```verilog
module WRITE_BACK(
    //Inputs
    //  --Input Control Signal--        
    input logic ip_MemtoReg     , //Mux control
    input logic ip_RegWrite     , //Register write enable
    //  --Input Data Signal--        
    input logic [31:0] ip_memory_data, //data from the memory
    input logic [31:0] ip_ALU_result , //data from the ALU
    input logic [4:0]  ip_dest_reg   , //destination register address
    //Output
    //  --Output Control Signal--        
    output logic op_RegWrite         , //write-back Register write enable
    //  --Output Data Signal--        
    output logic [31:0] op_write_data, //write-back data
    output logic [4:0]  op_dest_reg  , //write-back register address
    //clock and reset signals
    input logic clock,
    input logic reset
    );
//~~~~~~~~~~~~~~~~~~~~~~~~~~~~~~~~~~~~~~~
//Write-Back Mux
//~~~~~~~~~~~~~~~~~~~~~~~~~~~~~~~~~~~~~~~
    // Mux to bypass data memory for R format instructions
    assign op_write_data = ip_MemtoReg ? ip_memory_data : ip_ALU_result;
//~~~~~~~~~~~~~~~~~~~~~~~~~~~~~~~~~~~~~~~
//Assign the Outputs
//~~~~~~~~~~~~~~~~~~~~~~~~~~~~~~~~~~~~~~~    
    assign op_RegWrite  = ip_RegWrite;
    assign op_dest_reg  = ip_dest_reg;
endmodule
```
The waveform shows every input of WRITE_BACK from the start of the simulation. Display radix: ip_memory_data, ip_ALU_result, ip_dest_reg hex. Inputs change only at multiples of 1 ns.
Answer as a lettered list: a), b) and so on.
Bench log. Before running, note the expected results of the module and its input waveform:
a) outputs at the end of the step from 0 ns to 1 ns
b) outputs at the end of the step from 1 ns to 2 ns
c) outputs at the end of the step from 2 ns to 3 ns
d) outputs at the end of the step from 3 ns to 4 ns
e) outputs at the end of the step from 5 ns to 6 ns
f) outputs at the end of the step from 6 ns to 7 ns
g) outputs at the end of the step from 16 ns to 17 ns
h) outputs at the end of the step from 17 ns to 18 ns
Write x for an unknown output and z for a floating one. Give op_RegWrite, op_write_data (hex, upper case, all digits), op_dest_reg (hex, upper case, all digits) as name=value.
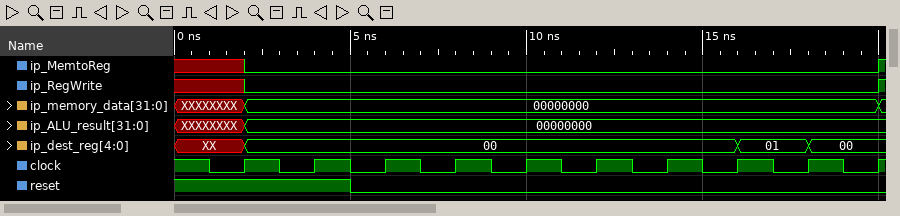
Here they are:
a) op_RegWrite=x, op_write_data=x, op_dest_reg=x
b) op_RegWrite=x, op_write_data=x, op_dest_reg=x
c) op_RegWrite=0, op_write_data=00000000, op_dest_reg=00
d) op_RegWrite=0, op_write_data=00000000, op_dest_reg=00
e) op_RegWrite=0, op_write_data=00000000, op_dest_reg=00
f) op_RegWrite=0, op_write_data=00000000, op_dest_reg=00
g) op_RegWrite=0, op_write_data=00000000, op_dest_reg=01
h) op_RegWrite=0, op_write_data=00000000, op_dest_reg=01
